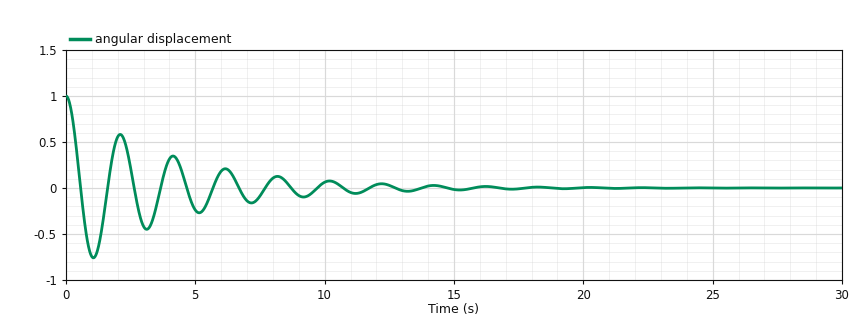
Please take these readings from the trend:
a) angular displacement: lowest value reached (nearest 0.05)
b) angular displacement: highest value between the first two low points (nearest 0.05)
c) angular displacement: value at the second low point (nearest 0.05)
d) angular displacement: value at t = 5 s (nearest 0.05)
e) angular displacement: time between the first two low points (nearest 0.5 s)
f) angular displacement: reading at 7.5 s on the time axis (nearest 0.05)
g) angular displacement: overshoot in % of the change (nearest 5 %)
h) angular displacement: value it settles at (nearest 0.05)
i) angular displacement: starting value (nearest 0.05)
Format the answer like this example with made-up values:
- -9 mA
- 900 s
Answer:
- -0.75
- 0.60
- -0.45
- -0.25
- 2.0 s
- -0.10
- 75 %
- 0.00
- 1.00
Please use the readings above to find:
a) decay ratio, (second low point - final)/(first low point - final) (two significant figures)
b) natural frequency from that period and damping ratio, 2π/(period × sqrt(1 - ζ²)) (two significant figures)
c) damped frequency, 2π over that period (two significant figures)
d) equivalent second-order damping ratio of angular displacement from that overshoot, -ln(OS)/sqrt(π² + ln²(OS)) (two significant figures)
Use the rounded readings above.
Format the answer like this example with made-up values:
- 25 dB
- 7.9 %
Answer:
- 0.60
- 3.2 rad/s
- 3.1 rad/s
- 0.091
